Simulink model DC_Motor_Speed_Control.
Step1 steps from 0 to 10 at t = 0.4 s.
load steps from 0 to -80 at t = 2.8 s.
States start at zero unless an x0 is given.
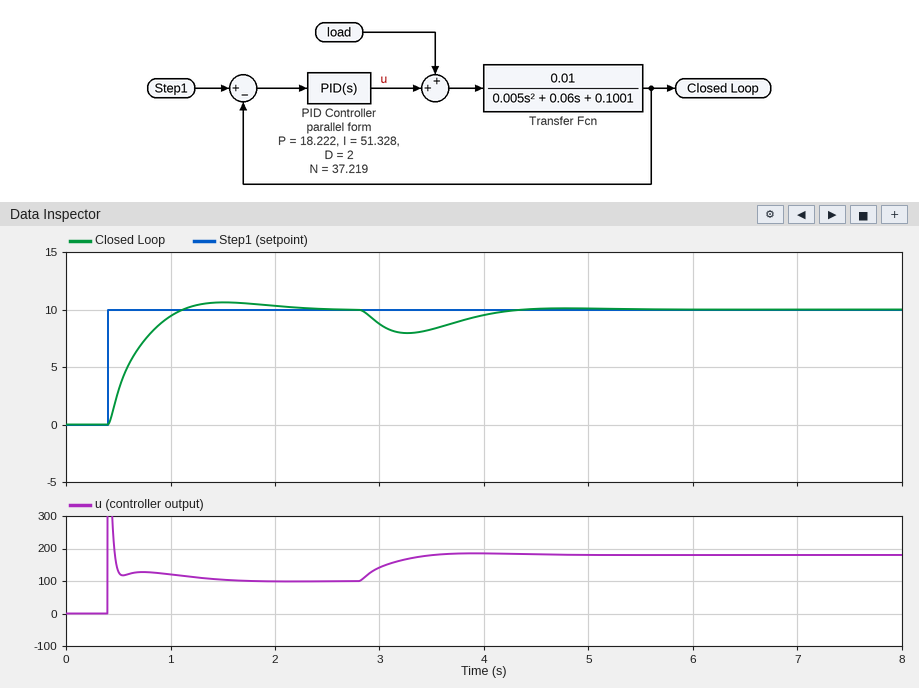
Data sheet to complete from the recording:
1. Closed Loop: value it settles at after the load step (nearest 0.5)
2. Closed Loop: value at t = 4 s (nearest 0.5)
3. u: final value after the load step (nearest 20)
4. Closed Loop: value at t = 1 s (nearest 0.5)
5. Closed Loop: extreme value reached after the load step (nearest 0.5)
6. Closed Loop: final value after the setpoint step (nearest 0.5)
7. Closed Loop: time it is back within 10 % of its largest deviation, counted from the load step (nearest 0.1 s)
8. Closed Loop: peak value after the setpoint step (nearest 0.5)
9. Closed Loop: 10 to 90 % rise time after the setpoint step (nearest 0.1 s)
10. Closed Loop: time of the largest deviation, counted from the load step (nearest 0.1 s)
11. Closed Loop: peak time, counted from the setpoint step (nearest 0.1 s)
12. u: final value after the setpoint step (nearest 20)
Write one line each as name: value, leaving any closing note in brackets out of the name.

Closed Loop: value it settles at after the load step: 10.0
Closed Loop: value at t = 4 s: 9.5
u: final value after the load step: 180
Closed Loop: value at t = 1 s: 9.5
Closed Loop: extreme value reached after the load step: 8.0
Closed Loop: final value after the setpoint step: 10.0
Closed Loop: time it is back within 10 % of its largest deviation, counted from the load step: 1.4 s
Closed Loop: peak value after the setpoint step: 10.5
Closed Loop: 10 to 90 % rise time after the setpoint step: 0.5 s
Closed Loop: time of the largest deviation, counted from the load step: 0.5 s
Closed Loop: peak time, counted from the setpoint step: 1.1 s
u: final value after the setpoint step: 100
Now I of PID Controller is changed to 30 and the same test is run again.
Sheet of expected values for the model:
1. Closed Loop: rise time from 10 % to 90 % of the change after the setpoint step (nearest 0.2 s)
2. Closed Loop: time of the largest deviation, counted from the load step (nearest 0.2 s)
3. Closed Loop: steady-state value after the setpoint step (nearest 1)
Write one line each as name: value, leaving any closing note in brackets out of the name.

Closed Loop: rise time from 10 % to 90 % of the change after the setpoint step: 0.8 s
Closed Loop: time of the largest deviation, counted from the load step: 0.6 s
Closed Loop: steady-state value after the setpoint step: 10
